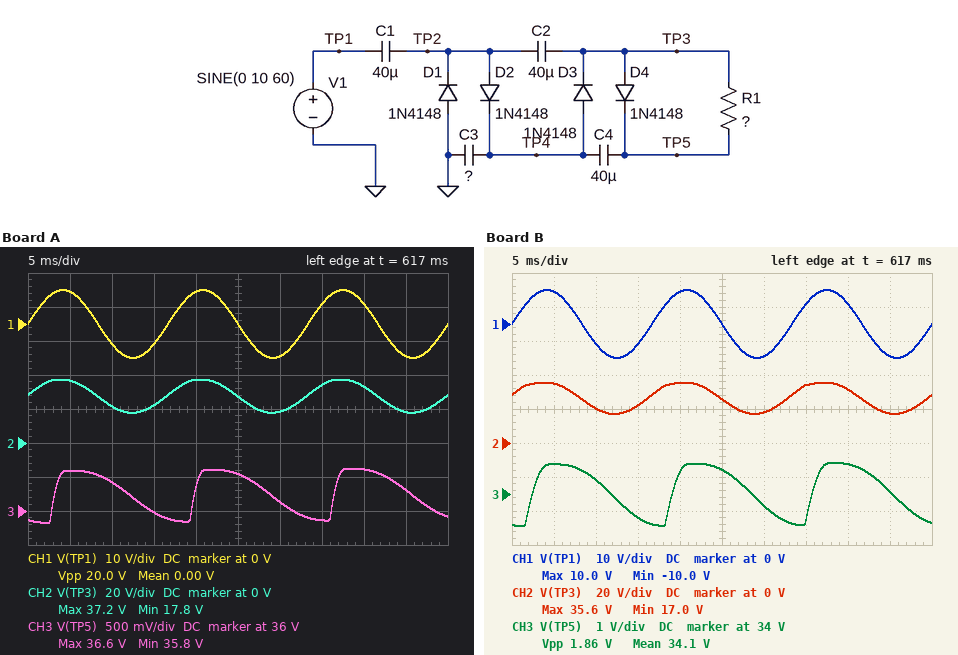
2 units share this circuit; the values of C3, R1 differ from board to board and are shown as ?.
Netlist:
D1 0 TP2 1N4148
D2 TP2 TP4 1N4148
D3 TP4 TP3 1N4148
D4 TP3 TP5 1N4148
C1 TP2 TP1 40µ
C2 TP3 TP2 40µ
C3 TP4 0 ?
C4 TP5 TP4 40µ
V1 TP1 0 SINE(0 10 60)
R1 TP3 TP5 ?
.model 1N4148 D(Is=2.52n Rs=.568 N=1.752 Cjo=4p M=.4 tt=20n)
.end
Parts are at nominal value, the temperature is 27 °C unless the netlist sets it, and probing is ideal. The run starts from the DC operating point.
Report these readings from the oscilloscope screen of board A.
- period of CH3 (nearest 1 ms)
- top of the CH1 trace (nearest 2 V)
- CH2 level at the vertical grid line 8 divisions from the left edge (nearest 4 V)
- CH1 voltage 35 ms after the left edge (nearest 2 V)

17 ms
10 V
32 V
6 V
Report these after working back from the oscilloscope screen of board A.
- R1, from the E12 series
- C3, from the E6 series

6.8 kΩ
100 µF
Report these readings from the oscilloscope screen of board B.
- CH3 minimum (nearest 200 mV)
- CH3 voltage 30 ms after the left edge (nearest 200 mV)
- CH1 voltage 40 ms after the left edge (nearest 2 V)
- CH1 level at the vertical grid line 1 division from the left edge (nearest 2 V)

33.0 V
33.6 V
6 V
10 V
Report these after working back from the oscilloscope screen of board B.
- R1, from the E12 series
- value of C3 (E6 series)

2.2 kΩ
150 µF
